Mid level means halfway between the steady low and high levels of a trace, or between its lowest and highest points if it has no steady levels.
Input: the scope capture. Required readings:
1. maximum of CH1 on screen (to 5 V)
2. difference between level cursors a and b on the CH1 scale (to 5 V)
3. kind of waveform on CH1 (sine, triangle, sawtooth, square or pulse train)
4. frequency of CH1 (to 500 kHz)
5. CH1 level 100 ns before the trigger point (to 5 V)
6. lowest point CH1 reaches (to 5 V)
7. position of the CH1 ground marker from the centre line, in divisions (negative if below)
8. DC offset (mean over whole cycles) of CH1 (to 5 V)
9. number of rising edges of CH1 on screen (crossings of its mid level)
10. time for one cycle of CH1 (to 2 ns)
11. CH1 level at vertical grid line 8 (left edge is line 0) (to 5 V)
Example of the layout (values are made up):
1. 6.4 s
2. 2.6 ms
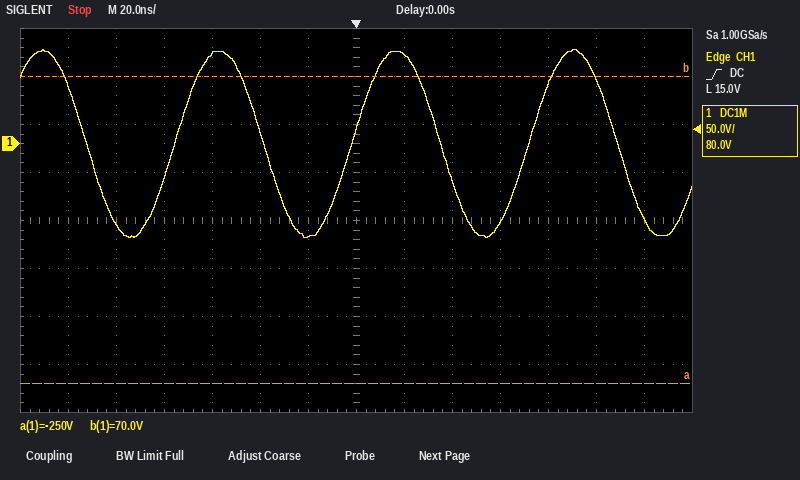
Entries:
1. 100 V
2. 320 V
3. sine
4. 13.5 MHz
5. -85 V
6. -100 V
7. +1.6 div
8. 0 V
9. 3
10. 74 ns
11. 95 V
